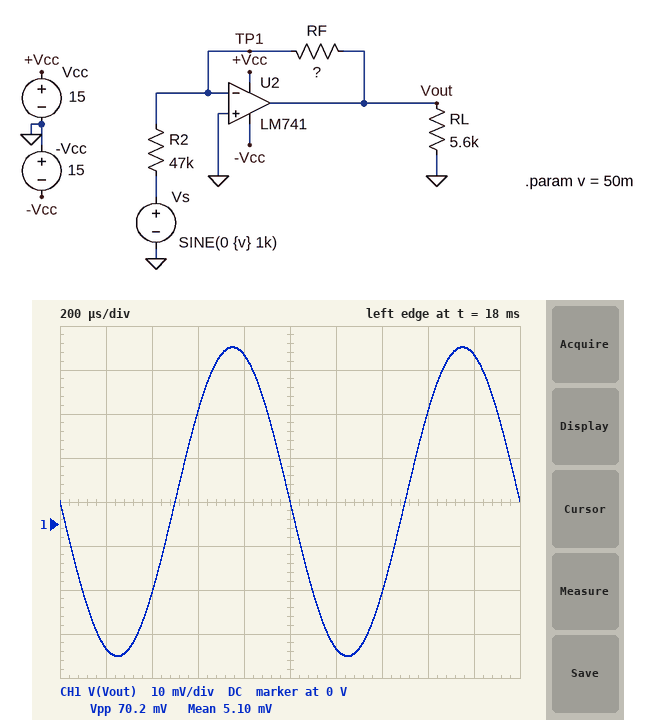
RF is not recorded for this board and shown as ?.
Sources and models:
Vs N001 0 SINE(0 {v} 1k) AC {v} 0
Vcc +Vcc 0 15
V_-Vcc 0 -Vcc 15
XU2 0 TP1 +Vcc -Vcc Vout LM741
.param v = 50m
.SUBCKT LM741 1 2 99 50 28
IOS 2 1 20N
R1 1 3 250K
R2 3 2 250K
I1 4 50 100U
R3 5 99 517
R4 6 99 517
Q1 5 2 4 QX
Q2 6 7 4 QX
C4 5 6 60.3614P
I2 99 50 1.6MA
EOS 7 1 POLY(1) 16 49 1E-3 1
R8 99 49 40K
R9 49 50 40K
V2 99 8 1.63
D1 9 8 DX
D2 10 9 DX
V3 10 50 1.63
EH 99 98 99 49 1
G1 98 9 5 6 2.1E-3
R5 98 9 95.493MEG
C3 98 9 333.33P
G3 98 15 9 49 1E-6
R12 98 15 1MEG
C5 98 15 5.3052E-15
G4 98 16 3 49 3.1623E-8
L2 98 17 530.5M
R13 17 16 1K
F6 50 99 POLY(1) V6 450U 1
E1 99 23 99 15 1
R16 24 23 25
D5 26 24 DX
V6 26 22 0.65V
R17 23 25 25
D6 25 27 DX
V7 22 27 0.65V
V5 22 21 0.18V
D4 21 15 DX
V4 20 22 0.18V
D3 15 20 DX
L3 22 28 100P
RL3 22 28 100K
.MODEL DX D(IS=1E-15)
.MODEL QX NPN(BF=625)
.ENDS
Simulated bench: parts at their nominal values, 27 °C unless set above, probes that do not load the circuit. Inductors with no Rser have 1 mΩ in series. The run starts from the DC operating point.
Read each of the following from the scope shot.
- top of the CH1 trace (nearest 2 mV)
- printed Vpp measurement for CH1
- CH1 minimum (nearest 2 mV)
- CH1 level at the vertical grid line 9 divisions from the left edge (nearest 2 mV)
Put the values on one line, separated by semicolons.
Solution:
40 mV; 70.2 mV; -30 mV; 38 mV
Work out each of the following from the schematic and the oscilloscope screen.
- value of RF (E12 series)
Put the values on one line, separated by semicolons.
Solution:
33 kΩ
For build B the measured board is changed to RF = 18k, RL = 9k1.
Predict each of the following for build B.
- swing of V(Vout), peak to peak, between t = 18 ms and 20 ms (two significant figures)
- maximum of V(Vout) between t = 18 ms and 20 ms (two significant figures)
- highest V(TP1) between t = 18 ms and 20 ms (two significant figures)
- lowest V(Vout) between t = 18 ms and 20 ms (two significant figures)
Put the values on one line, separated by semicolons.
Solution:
38 mV; 22 mV; 1.0 mV; -16 mV
